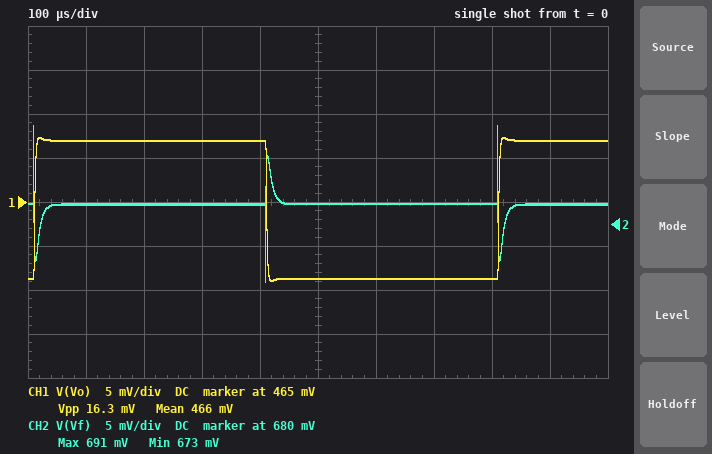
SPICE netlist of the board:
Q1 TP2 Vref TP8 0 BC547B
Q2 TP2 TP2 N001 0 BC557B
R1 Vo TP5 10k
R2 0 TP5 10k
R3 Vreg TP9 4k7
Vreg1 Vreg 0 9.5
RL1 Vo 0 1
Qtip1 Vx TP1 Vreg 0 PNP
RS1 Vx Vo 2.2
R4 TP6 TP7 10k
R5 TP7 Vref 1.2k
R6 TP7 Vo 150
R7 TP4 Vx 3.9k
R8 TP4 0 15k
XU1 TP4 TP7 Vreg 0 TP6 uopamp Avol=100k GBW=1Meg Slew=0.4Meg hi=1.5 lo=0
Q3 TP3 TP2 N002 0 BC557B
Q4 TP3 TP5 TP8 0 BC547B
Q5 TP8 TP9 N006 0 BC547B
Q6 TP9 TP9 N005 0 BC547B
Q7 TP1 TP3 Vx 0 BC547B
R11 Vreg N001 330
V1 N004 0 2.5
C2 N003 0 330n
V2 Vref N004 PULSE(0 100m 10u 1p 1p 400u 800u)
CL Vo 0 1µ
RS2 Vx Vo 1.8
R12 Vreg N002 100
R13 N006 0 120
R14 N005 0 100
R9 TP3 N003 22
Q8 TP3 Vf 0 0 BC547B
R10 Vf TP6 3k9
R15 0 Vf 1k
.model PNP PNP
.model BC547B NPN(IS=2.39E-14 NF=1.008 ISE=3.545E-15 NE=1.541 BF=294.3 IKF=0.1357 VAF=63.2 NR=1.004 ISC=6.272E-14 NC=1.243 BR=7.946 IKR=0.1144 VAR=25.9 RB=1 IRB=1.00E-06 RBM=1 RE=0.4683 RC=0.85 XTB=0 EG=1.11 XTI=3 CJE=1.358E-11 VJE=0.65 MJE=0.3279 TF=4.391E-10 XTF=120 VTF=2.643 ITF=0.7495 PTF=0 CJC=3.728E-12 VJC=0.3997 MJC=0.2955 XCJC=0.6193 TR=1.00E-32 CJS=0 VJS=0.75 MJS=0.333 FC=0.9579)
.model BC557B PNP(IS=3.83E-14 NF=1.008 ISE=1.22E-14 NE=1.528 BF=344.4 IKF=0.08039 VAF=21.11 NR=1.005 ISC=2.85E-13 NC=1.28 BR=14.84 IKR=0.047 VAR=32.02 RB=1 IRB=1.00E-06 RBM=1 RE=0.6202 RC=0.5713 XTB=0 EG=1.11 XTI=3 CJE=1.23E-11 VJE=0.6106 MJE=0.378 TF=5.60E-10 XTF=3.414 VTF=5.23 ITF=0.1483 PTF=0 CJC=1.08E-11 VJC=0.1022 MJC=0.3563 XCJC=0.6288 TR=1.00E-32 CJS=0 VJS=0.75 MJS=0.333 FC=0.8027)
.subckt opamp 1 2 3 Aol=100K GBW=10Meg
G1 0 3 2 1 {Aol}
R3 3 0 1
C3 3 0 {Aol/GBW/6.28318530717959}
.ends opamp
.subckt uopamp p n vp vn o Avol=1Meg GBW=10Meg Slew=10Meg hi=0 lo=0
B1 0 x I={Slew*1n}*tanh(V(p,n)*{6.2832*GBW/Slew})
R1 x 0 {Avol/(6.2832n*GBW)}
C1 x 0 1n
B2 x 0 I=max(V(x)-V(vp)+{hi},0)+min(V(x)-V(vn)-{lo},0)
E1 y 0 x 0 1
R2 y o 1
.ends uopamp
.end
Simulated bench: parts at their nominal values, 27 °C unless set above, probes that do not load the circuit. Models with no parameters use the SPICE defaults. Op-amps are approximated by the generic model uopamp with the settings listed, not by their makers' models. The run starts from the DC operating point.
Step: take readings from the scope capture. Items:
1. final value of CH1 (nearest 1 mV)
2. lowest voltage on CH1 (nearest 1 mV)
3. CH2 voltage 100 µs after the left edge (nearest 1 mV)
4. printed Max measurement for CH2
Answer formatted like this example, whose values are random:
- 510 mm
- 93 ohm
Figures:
- 472 mV
- 456 mV
- 682 mV
- 691 mV
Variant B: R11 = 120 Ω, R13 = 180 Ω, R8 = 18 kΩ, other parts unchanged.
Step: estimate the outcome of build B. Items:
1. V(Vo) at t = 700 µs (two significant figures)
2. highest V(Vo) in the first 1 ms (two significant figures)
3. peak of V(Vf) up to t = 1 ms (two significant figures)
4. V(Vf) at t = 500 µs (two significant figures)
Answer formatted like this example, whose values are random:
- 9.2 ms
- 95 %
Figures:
- 420 mV
- 430 mV
- 660 mV
- 650 mV
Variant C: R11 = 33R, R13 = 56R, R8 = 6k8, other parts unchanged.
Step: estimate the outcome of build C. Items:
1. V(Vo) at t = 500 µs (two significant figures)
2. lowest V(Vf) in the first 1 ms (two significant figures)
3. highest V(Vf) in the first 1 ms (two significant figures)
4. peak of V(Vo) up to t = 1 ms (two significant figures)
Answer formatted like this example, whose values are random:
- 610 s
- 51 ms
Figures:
- 820 mV
- 610 mV
- 660 mV
- 850 mV
